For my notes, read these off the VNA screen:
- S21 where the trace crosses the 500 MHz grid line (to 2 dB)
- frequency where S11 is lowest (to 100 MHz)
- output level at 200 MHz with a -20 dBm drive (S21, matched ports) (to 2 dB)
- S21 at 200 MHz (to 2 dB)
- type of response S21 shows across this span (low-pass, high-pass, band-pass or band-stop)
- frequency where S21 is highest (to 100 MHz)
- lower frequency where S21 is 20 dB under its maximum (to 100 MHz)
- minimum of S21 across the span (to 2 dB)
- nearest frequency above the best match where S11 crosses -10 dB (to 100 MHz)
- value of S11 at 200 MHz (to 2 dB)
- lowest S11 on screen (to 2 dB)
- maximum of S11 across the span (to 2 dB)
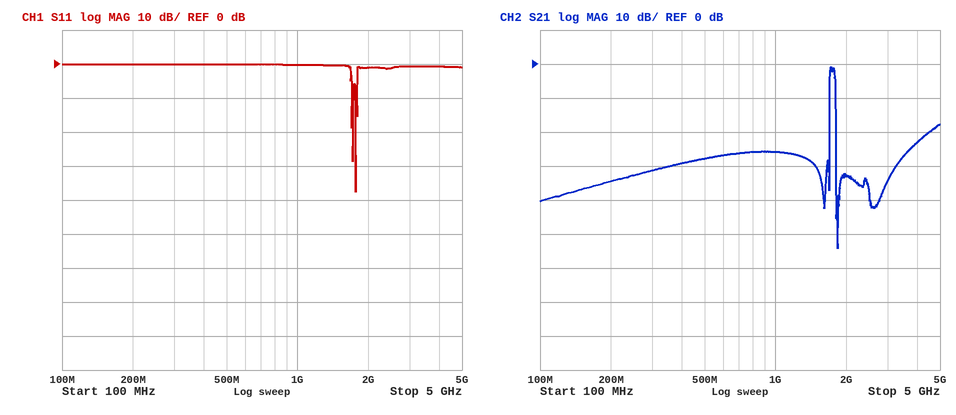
-28 dB
1.8 GHz
-54 dBm
-34 dB
band-pass
1.7 GHz
1.7 GHz
-54 dB
1.8 GHz
0 dB
-38 dB
0 dB
